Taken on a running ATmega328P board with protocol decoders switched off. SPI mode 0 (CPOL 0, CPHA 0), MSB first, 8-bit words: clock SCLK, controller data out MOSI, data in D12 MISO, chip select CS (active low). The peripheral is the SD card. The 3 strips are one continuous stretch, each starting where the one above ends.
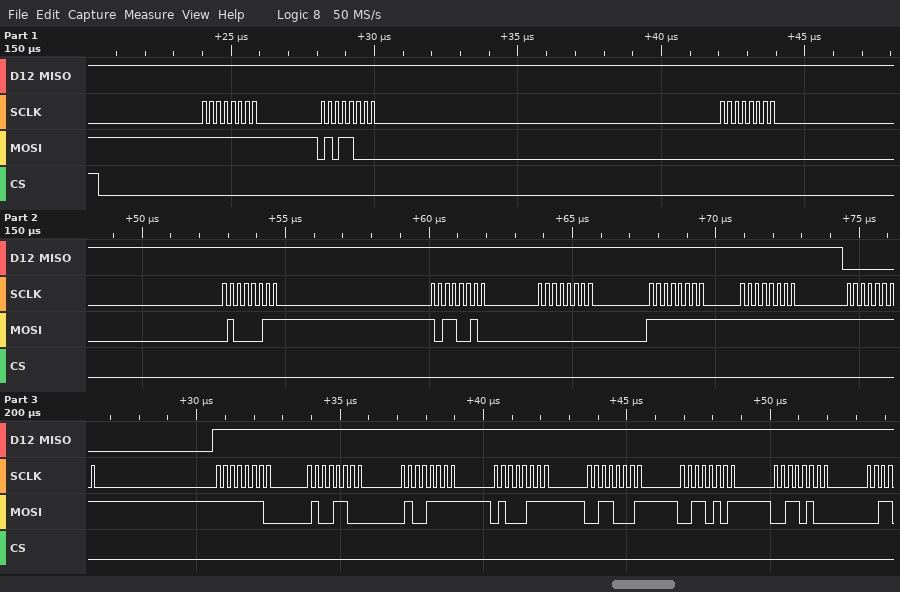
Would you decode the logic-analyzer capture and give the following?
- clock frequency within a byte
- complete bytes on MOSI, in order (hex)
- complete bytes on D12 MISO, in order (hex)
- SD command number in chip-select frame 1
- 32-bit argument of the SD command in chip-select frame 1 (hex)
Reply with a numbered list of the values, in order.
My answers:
1. 4 MHz
2. FF 58 00 43 B2 00 FF FF FF FE 4C 4F 47 31 35 34
3. FF FF FF FF FF FF FF FF 00 FF FF FF FF FF FF FF
4. CMD24
5. 0x0043B200
